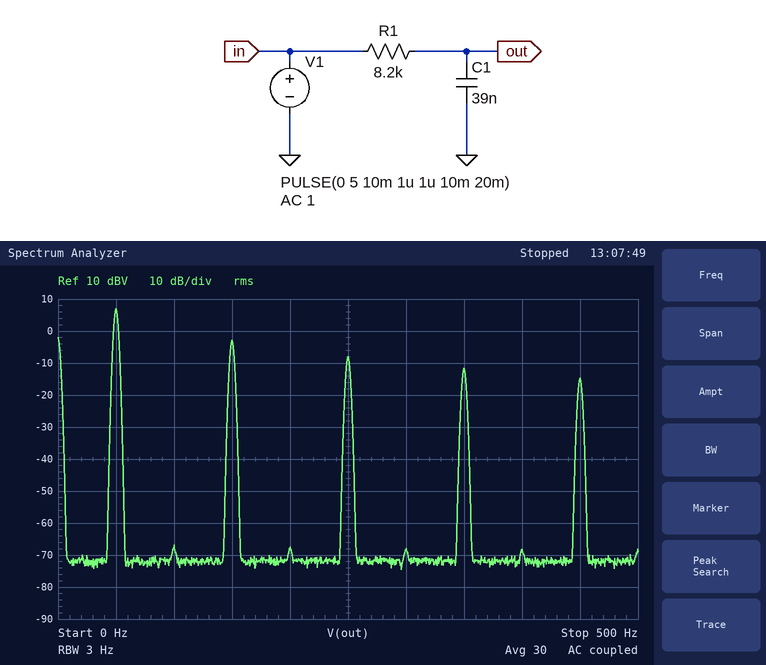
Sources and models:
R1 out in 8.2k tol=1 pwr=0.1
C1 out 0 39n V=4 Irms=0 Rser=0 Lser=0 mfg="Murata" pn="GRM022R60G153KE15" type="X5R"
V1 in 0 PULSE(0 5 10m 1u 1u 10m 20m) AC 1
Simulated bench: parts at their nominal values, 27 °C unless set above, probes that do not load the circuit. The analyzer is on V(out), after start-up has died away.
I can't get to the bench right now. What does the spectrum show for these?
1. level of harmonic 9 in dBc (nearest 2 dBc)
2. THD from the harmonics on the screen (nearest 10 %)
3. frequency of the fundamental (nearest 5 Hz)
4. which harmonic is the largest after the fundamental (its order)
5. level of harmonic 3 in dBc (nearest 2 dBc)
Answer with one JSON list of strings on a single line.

["-22 dBc", "40 %", "50 Hz", "3", "-10 dBc"]
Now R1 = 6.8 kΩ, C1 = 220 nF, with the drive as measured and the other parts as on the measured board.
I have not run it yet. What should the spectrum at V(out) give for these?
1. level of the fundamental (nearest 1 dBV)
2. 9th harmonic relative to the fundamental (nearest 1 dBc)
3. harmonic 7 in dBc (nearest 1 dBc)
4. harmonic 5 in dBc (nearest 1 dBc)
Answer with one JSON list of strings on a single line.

["6 dBV", "-31 dBc", "-27 dBc", "-21 dBc"]
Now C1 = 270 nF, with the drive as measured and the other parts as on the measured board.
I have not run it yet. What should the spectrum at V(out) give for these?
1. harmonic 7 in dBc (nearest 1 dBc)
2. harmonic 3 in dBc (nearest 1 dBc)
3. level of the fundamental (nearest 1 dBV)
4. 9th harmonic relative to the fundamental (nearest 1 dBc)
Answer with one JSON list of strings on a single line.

["-29 dBc", "-15 dBc", "5 dBV", "-33 dBc"]
